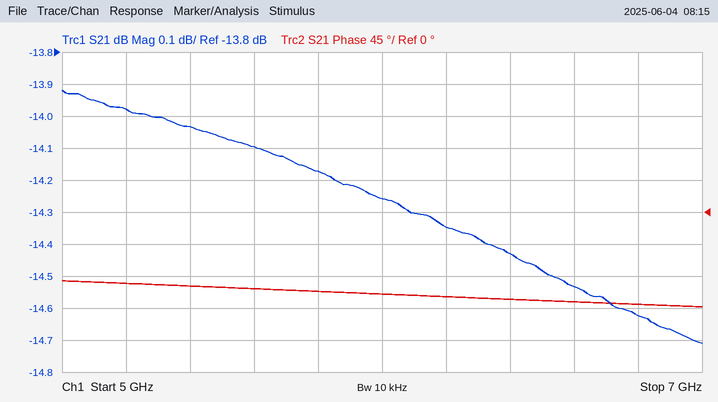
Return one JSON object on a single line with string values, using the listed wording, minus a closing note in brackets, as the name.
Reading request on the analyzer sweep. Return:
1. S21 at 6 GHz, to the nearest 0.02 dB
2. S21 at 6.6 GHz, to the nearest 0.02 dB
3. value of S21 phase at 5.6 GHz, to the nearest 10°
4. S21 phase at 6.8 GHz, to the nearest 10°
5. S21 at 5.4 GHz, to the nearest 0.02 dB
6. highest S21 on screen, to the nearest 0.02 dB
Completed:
{"S21 at 6 GHz, to the nearest 0.02 dB": "-14.26 dB", "S21 at 6.6 GHz, to the nearest 0.02 dB": "-14.54 dB", "value of S21 phase at 5.6 GHz, to the nearest 10°": "-110°", "S21 phase at 6.8 GHz, to the nearest 10°": "-130°", "S21 at 5.4 GHz, to the nearest 0.02 dB": "-14.04 dB", "highest S21 on screen, to the nearest 0.02 dB": "-13.92 dB"}
